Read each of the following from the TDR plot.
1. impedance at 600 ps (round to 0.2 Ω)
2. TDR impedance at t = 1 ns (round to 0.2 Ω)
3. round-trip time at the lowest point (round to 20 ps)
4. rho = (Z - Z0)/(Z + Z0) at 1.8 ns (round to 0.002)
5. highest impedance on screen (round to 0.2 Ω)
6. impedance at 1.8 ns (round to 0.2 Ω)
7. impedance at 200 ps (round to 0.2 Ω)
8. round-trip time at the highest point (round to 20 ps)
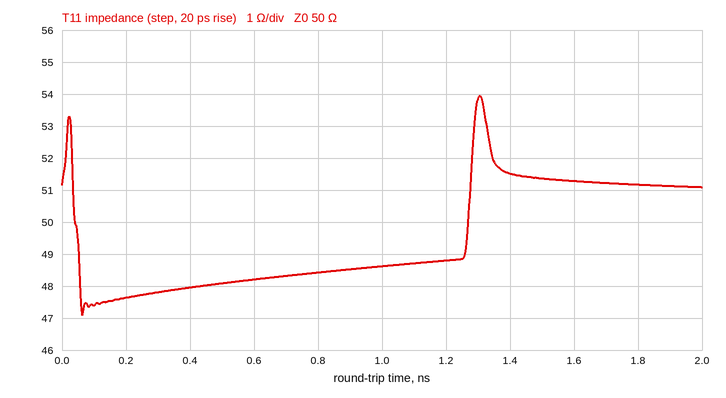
48.2 Ω
48.6 Ω
60 ps
+0.012
54.0 Ω
51.2 Ω
47.6 Ω
1.30 ns
